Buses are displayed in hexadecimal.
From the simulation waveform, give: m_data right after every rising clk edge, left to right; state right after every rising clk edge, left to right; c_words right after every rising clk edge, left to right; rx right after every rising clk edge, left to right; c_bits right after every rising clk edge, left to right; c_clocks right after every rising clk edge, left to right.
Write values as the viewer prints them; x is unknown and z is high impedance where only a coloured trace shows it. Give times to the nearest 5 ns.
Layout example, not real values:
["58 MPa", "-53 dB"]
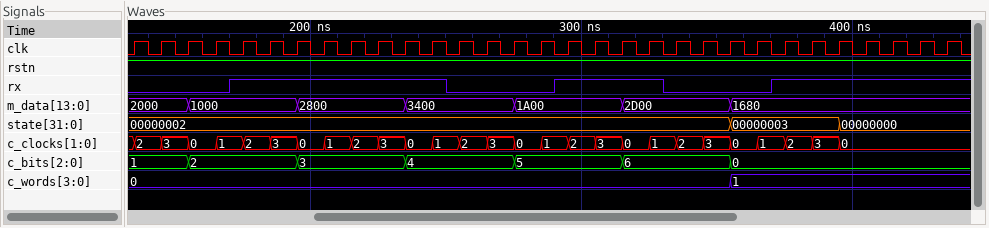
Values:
["2000, 2000, 1000, 1000, 1000, 1000, 2800, 2800, 2800, 2800, 3400, 3400, 3400, 3400, 1A00, 1A00, 1A00, 1A00, 2D00, 2D00, 2D00, 2D00, 1680, 1680, 1680, 1680, 1680, 1680, 1680, 1680, 1680", "00000002, 00000002, 00000002, 00000002, 00000002, 00000002, 00000002, 00000002, 00000002, 00000002, 00000002, 00000002, 00000002, 00000002, 00000002, 00000002, 00000002, 00000002, 00000002, 00000002, 00000002, 00000002, 00000003, 00000003, 00000003, 00000003, 00000000, 00000000, 00000000, 00000000, 00000000", "0, 0, 0, 0, 0, 0, 0, 0, 0, 0, 0, 0, 0, 0, 0, 0, 0, 0, 0, 0, 0, 0, 1, 1, 1, 1, 1, 1, 1, 1, 1", "0 0 0 0 1 1 1 1 1 1 1 1 0 0 0 0 1 1 1 1 0 0 0 0 1 1 1 1 1 1 1", "1, 1, 2, 2, 2, 2, 3, 3, 3, 3, 4, 4, 4, 4, 5, 5, 5, 5, 6, 6, 6, 6, 0, 0, 0, 0, 0, 0, 0, 0, 0", "2, 3, 0, 1, 2, 3, 0, 1, 2, 3, 0, 1, 2, 3, 0, 1, 2, 3, 0, 1, 2, 3, 0, 1, 2, 3, 0, 0, 0, 0, 0"]
